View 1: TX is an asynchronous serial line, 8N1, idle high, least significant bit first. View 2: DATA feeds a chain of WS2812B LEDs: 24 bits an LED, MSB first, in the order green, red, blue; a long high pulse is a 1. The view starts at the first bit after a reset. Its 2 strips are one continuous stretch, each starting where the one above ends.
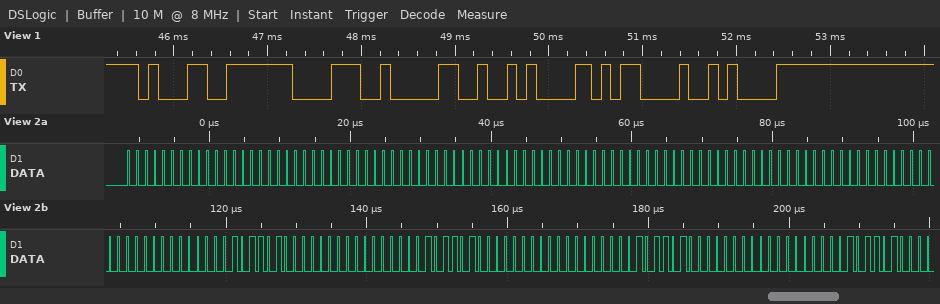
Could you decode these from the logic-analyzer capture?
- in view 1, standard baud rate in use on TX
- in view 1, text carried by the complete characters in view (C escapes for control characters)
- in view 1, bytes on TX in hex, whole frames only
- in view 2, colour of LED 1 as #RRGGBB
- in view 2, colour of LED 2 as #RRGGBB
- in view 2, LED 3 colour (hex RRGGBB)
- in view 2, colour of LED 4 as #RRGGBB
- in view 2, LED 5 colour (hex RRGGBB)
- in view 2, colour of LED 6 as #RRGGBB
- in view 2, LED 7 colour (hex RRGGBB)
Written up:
9600 baud
"180\n\r\n"
0x31 0x38 0x30 0x0A 0x0D 0x0A
#000000
#000000
#000000
#000000
#2D0000
#B40000
#B40000
